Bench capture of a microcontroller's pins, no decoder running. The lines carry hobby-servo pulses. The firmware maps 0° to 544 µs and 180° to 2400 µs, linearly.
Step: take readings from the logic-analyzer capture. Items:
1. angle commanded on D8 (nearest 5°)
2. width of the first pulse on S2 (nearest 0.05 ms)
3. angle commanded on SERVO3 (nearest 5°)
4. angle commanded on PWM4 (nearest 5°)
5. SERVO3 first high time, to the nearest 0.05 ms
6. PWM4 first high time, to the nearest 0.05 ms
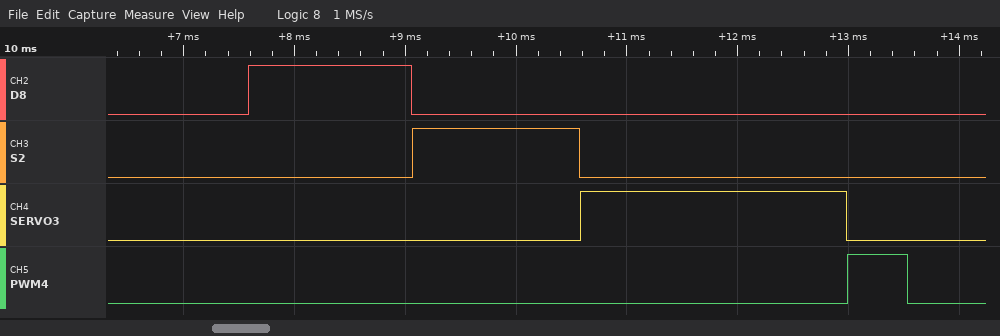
90°
1.50 ms
180°
0°
2.40 ms
0.55 ms
